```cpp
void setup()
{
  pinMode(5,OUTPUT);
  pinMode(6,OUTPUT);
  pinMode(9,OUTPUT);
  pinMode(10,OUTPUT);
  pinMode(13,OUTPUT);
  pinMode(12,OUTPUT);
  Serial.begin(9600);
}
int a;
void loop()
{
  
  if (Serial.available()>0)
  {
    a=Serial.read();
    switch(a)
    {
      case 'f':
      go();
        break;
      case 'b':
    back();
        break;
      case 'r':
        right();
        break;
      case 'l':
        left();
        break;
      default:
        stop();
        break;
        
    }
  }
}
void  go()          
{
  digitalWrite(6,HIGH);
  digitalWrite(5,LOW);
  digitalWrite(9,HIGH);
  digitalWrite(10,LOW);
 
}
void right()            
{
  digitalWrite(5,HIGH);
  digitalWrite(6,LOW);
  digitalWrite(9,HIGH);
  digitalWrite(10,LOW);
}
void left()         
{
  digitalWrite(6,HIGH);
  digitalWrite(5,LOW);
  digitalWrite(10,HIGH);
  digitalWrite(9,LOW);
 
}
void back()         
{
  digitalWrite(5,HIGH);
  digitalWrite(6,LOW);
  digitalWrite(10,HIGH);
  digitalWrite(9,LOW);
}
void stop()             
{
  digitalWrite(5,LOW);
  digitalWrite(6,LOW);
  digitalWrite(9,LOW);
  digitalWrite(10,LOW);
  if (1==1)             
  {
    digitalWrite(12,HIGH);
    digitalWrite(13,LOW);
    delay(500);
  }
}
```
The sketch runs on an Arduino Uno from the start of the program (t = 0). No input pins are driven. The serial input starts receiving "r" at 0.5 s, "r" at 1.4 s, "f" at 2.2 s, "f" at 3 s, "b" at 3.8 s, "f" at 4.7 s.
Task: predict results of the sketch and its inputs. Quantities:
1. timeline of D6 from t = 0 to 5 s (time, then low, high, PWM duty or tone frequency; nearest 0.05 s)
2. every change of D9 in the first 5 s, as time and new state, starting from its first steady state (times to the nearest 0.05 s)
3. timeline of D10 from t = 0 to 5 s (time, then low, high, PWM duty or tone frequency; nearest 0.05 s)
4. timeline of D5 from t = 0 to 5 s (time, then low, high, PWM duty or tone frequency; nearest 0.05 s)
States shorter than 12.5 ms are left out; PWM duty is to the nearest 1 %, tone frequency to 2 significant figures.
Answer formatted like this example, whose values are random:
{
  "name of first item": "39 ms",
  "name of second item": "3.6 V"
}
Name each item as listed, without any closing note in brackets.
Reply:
{
  "timeline of D6 from t = 0 to 5 s": "0 s low; 2.2 s high; 3.8 s low; 4.7 s high",
  "every change of D9 in the first 5 s, as time and new state, starting from its first steady state": "0 s low; 0.5 s high; 3.8 s low; 4.7 s high",
  "timeline of D10 from t = 0 to 5 s": "0 s low; 3.8 s high; 4.7 s low",
  "timeline of D5 from t = 0 to 5 s": "0 s low; 0.5 s high; 2.2 s low; 3.8 s high; 4.7 s low"
}
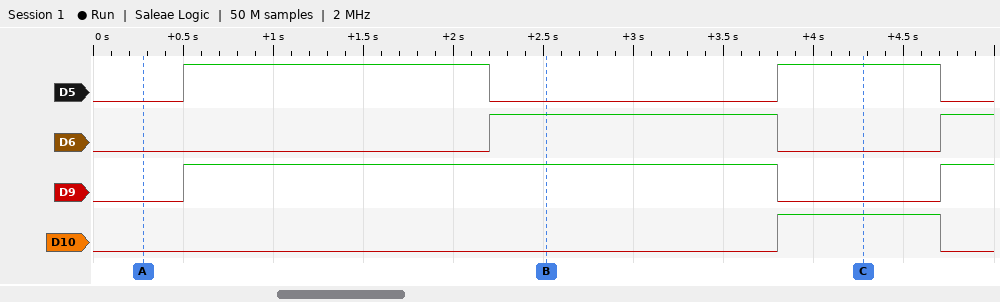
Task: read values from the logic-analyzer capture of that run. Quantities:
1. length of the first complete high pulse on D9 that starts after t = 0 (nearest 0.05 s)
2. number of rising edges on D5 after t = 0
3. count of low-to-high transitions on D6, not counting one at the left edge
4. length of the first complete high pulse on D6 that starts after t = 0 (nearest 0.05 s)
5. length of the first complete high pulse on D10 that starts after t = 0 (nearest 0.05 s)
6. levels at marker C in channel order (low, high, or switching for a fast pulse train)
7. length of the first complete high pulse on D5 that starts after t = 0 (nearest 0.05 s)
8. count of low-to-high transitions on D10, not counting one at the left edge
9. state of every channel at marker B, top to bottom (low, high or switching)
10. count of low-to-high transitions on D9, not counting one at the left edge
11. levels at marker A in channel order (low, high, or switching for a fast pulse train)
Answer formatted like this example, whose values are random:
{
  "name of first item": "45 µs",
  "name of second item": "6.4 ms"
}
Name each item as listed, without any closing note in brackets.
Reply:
{
  "length of the first complete high pulse on D9 that starts after t = 0": "3.30 s",
  "number of rising edges on D5 after t = 0": "2",
  "count of low-to-high transitions on D6, not counting one at the left edge": "2",
  "length of the first complete high pulse on D6 that starts after t = 0": "1.60 s",
  "length of the first complete high pulse on D10 that starts after t = 0": "0.90 s",
  "levels at marker C in channel order": "D5 high, D6 low, D9 low, D10 high",
  "length of the first complete high pulse on D5 that starts after t = 0": "1.70 s",
  "count of low-to-high transitions on D10, not counting one at the left edge": "1",
  "state of every channel at marker B, top to bottom": "D5 low, D6 high, D9 high, D10 low",
  "count of low-to-high transitions on D9, not counting one at the left edge": "2",
  "levels at marker A in channel order": "D5 low, D6 low, D9 low, D10 low"
}
